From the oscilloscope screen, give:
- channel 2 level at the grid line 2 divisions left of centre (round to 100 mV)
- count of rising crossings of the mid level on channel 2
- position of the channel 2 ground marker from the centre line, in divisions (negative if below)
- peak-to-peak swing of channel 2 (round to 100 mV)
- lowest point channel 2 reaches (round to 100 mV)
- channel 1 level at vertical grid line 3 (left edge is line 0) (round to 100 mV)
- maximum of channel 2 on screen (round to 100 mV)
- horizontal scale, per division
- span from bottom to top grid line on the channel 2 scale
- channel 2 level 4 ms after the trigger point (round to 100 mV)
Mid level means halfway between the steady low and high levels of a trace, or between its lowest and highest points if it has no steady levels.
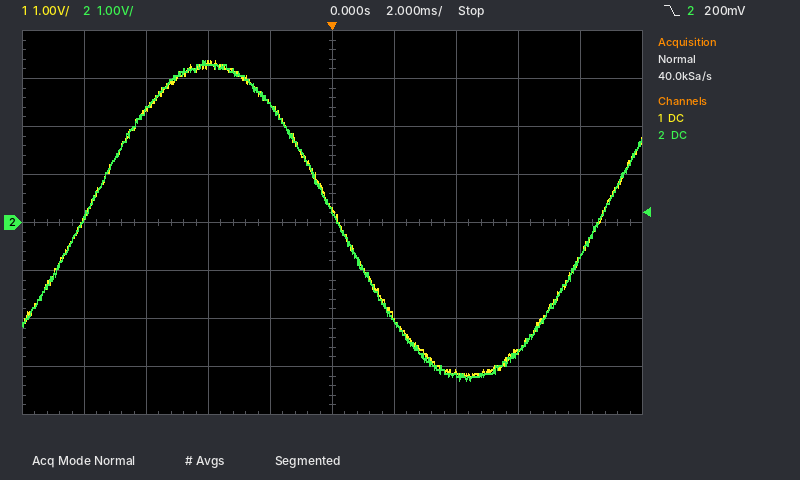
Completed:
3.3 V
2
0.0 div
6.7 V
-3.3 V
3.3 V
3.4 V
2 ms
8 V
-3.2 V
